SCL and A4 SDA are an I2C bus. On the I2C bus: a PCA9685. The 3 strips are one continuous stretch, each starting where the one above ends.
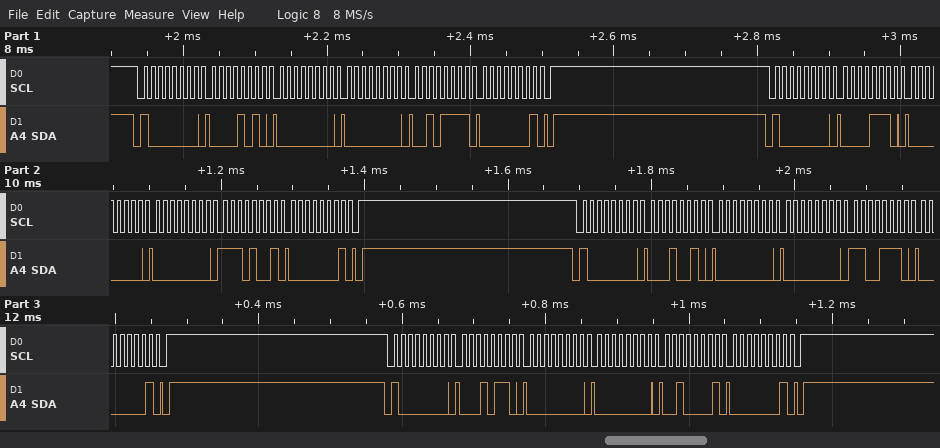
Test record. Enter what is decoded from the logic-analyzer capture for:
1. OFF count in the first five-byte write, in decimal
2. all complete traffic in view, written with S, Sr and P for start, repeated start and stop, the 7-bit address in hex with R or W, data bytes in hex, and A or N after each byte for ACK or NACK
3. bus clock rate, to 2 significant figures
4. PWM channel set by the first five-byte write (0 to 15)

303
S 40W A 0A A 00 A 00 A 2F A 01 A P S 40W A 0E A 00 A 00 A E9 A 01 A P S 40W A 12 A 00 A 00 A CE A 01 A P S 40W A 16 A 00 A 00 A 21 A 01 A P
100 kHz
1
